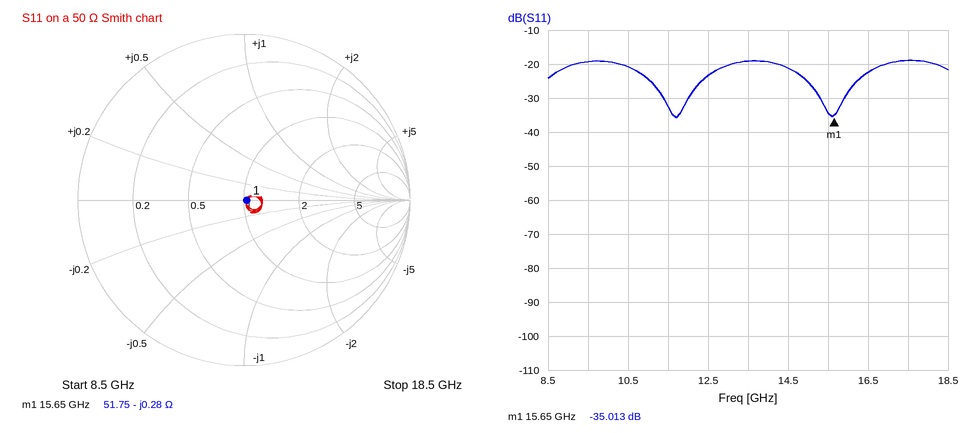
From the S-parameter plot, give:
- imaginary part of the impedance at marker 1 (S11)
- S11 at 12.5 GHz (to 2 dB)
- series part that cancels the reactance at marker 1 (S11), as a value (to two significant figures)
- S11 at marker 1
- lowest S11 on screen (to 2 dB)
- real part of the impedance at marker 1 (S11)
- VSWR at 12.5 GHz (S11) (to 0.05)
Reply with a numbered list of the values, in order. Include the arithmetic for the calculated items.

1. -0.28 Ω
2. -24 dB
3. L = 0.28 Ω/(2π × 15.65 GHz) ≈ 2.8 pH
4. -35.013 dB
5. -36 dB
6. 51.75 Ω
7. |Γ| = 10^(-24/20) = 0.0631; VSWR = (1 + 0.0631)/(1 − 0.0631) ≈ 1.13, so 1.15 to the nearest 0.05
